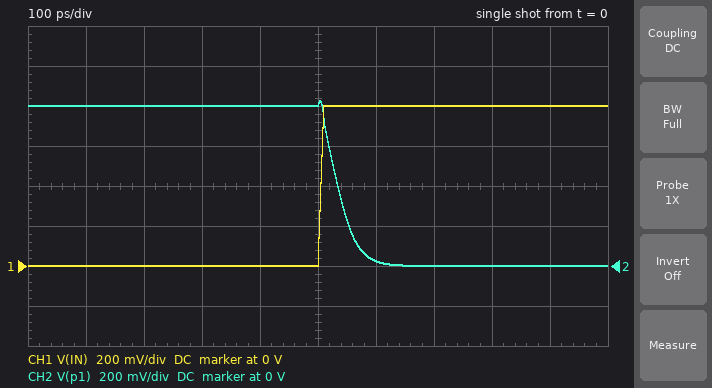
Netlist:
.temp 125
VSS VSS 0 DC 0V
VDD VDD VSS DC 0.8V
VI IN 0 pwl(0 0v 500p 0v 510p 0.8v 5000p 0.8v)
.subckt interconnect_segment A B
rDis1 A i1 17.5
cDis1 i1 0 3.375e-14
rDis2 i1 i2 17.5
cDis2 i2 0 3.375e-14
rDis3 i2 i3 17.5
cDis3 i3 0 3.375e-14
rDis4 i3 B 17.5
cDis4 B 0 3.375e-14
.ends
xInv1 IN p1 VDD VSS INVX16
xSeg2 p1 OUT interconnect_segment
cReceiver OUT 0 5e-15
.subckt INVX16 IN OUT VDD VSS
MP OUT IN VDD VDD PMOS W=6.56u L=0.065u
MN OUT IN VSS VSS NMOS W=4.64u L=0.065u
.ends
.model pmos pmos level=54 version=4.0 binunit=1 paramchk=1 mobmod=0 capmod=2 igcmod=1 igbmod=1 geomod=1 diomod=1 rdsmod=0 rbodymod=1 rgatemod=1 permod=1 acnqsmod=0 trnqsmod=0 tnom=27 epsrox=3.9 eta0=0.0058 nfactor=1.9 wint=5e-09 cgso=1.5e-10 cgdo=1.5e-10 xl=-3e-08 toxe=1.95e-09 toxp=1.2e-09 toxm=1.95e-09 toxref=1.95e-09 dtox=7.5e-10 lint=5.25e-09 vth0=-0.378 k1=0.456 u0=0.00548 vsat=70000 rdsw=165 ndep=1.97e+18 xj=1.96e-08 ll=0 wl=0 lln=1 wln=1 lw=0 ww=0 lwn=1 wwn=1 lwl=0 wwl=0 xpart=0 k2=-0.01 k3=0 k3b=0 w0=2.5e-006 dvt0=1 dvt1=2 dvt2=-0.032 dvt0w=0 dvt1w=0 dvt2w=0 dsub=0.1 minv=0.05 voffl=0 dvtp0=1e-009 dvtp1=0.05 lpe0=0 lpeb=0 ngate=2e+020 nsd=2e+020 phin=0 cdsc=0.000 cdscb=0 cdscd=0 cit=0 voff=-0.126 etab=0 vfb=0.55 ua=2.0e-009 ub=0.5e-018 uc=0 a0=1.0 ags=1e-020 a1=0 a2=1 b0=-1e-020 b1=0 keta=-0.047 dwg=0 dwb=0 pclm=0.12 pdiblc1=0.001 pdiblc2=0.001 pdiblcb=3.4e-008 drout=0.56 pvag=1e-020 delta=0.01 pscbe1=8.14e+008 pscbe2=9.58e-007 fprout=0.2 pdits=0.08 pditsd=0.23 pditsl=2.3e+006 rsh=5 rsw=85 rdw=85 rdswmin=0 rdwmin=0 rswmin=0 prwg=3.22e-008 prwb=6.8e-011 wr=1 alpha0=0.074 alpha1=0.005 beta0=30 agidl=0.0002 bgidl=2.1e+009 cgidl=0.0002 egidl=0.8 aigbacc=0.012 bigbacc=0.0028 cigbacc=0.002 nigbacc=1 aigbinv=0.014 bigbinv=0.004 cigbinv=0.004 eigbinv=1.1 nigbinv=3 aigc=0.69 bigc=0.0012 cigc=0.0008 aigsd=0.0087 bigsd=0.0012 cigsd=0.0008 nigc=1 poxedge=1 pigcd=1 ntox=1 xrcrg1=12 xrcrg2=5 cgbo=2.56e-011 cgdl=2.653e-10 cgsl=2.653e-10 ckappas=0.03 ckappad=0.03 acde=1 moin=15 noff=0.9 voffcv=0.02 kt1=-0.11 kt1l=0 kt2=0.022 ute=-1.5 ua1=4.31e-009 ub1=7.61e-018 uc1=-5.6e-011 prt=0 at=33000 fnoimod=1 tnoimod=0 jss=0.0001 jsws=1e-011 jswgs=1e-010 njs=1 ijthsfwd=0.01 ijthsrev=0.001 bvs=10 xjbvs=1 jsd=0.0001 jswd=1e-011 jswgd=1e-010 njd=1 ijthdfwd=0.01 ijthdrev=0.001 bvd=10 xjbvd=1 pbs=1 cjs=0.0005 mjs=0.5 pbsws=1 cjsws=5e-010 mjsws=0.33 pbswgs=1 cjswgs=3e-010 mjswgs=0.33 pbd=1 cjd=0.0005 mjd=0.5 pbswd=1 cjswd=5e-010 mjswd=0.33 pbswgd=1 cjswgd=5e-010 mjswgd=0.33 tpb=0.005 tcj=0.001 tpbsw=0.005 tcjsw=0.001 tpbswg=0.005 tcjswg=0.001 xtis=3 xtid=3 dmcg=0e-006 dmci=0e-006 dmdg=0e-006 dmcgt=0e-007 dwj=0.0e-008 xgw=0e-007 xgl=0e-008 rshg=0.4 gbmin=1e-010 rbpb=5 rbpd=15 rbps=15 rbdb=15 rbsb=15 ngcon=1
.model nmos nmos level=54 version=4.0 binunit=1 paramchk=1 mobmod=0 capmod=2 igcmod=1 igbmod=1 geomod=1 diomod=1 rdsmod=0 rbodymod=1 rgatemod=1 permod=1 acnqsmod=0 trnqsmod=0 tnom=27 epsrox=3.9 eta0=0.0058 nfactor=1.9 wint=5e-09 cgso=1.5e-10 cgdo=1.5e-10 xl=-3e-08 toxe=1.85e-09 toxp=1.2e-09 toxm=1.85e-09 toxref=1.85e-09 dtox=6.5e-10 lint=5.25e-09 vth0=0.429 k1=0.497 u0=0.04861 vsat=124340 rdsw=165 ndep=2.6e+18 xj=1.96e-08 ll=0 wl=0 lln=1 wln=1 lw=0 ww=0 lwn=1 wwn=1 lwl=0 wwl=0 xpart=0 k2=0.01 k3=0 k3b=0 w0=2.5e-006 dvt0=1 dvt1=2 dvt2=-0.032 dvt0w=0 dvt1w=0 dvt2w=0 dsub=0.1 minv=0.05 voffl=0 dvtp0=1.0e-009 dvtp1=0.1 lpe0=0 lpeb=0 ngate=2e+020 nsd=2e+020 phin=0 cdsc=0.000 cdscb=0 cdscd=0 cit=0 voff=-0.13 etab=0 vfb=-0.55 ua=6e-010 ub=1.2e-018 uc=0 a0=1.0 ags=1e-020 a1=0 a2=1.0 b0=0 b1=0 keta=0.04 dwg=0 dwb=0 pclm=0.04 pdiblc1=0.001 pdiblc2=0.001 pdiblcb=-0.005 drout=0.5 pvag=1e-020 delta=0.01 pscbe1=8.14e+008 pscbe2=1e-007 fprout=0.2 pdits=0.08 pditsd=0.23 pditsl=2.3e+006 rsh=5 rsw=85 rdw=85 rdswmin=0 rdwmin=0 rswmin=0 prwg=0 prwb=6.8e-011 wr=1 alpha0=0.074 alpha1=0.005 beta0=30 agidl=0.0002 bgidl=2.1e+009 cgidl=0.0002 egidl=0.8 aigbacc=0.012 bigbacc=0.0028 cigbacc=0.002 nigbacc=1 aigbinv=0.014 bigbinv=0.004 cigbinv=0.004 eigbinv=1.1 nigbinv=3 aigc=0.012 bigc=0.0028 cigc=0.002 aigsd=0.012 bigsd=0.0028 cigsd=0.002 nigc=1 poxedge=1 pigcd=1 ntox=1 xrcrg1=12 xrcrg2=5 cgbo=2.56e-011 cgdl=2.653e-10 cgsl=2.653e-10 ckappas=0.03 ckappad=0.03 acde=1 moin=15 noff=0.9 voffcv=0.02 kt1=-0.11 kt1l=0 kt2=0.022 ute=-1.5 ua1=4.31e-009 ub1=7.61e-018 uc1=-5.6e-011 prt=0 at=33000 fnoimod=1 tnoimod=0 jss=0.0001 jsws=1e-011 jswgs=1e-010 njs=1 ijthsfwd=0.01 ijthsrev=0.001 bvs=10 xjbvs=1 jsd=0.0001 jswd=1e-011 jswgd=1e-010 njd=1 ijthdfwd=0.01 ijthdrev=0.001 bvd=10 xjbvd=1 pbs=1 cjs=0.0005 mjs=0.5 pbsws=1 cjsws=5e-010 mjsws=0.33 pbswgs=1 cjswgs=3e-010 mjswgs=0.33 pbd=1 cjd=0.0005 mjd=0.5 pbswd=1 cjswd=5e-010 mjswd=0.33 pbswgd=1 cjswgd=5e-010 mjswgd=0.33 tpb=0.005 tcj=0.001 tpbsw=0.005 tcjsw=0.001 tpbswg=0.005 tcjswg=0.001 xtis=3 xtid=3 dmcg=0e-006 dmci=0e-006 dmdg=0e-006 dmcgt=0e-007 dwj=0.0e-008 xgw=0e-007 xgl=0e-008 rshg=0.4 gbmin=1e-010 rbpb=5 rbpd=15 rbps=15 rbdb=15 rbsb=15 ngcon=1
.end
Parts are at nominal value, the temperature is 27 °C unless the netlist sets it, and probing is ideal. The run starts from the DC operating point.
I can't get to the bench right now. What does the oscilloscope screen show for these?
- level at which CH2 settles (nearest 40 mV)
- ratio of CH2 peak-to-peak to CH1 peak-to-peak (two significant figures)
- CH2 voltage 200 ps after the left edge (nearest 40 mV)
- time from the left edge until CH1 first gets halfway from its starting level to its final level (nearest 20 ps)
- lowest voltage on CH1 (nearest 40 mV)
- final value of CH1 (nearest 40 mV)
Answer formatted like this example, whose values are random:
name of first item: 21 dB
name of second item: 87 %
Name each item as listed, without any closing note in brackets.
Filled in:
level at which CH2 settles: 0 V
ratio of CH2 peak-to-peak to CH1 peak-to-peak: 1.0
CH2 voltage 200 ps after the left edge: 800 mV
time from the left edge until CH1 first gets halfway from its starting level to its final level: 500 ps
lowest voltage on CH1: 0 V
final value of CH1: 800 mV
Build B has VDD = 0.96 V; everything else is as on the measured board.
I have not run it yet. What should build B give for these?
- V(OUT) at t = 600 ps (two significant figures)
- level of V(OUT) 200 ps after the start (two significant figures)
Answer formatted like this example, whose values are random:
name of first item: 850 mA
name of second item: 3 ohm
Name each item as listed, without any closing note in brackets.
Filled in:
V(OUT) at t = 600 ps: 54 mV
level of V(OUT) 200 ps after the start: 960 mV
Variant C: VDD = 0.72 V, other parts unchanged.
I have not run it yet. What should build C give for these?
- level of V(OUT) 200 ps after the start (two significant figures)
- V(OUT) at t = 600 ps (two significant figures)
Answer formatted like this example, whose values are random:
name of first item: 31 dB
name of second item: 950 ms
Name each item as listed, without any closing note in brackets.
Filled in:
level of V(OUT) 200 ps after the start: 720 mV
V(OUT) at t = 600 ps: 26 mV
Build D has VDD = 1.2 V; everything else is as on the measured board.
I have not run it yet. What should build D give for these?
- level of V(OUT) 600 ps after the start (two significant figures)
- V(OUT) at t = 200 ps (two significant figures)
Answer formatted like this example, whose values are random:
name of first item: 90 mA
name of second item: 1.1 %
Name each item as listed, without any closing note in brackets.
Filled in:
level of V(OUT) 600 ps after the start: 130 mV
V(OUT) at t = 200 ps: 1.2 V
